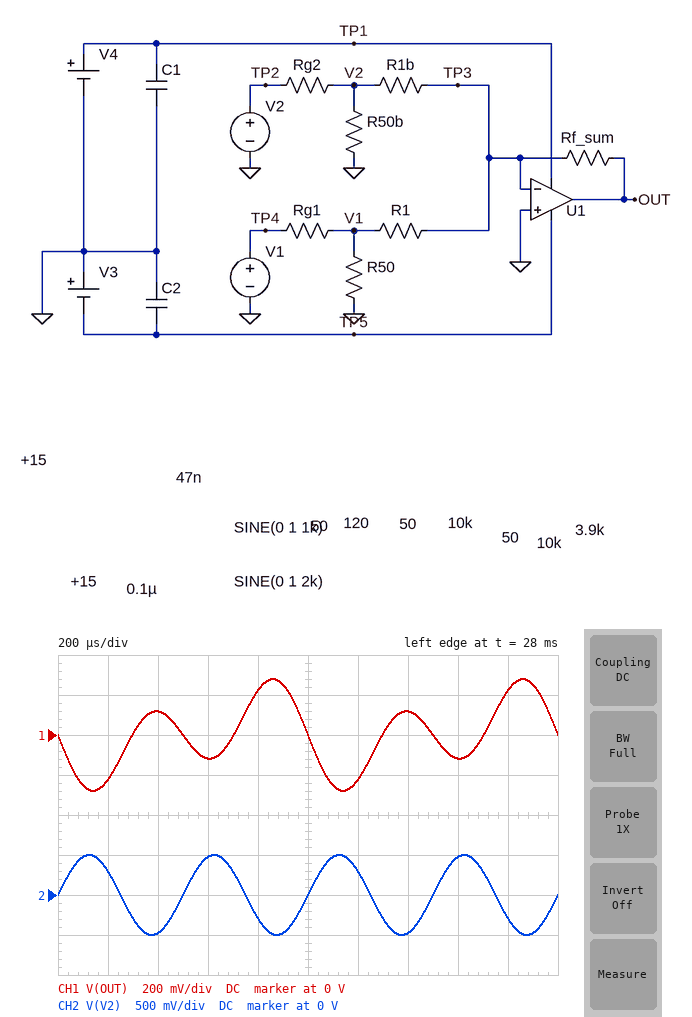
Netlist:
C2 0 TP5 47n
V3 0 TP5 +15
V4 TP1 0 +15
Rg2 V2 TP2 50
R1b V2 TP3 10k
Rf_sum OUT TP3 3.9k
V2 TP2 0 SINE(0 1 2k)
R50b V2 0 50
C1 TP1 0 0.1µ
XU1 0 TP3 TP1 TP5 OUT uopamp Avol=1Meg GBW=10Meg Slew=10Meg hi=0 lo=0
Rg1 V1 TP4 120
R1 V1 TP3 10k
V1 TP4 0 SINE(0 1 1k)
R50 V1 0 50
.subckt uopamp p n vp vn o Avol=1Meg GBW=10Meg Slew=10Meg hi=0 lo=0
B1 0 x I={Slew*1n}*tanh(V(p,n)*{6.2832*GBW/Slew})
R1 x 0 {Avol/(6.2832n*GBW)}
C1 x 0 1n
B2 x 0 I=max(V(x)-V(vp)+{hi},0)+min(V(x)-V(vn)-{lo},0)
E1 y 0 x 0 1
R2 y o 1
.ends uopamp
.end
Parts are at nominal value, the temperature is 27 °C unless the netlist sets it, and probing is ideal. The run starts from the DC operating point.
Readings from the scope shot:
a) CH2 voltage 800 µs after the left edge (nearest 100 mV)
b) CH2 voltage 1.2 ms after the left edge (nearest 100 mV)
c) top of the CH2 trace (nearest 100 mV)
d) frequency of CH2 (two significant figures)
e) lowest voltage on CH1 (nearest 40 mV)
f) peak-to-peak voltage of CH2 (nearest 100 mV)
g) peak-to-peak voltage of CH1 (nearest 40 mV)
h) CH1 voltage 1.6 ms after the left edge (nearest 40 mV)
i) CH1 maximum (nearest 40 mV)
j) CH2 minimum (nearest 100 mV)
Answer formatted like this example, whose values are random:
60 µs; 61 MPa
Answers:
-300 mV; 300 mV; 500 mV; 2.0 kHz; -280 mV; 1.0 V; 560 mV; -120 mV; 280 mV; -500 mV
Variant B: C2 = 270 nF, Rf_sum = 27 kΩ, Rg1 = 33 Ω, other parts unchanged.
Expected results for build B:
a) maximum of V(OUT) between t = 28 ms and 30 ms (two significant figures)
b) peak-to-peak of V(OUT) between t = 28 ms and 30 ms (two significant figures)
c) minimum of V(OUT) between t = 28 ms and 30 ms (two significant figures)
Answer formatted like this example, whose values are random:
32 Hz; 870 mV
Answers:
2.6 V; 5.2 V; -2.6 V
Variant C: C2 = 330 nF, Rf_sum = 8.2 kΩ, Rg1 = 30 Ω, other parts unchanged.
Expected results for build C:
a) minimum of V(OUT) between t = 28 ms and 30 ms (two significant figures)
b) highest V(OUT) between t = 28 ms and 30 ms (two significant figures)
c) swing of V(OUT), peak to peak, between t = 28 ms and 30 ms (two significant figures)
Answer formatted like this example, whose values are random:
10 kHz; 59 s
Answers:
-800 mV; 800 mV; 1.6 V
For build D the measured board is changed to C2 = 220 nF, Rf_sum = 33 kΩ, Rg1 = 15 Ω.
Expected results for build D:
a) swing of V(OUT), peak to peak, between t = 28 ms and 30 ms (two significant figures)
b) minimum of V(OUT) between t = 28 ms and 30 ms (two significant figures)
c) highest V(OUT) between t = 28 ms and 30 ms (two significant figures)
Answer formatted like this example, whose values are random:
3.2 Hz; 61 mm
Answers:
7.3 V; -3.6 V; 3.6 V
